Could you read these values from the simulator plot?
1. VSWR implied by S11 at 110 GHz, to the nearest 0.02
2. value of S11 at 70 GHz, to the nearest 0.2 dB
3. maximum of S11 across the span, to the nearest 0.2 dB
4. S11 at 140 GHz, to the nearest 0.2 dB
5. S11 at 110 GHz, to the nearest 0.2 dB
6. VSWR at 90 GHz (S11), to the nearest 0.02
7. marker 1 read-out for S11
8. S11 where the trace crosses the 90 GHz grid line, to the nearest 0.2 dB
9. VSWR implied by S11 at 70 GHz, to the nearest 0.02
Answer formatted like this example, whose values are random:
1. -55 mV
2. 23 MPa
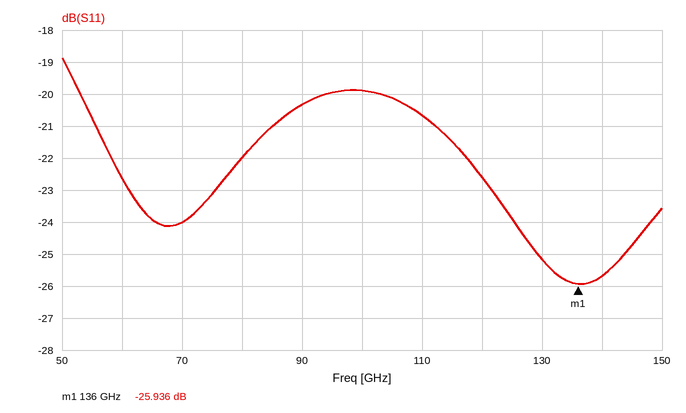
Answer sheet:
1. 1.20
2. -24.0 dB
3. -18.8 dB
4. -25.6 dB
5. -20.6 dB
6. 1.22
7. -25.936 dB
8. -20.4 dB
9. 1.14
